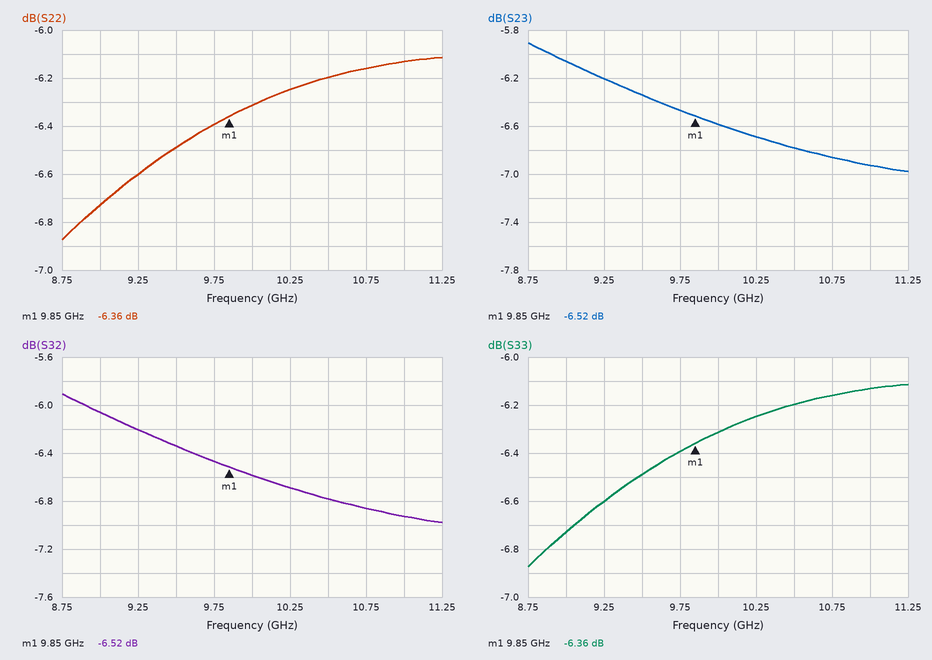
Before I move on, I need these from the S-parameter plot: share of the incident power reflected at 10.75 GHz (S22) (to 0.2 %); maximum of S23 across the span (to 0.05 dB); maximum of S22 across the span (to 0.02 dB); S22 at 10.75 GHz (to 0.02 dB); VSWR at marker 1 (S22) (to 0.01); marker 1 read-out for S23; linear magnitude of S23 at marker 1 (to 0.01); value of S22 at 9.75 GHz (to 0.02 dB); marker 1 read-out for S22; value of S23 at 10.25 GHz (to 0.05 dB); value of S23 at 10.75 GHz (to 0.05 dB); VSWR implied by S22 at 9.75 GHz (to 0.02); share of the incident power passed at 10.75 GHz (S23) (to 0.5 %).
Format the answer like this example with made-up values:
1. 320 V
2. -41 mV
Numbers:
1. 24.2 %
2. -5.90 dB
3. -6.12 dB
4. -6.16 dB
5. 2.85
6. -6.52 dB
7. 0.47
8. -6.40 dB
9. -6.36 dB
10. -6.70 dB
11. -6.85 dB
12. 2.84
13. 20.5 %
